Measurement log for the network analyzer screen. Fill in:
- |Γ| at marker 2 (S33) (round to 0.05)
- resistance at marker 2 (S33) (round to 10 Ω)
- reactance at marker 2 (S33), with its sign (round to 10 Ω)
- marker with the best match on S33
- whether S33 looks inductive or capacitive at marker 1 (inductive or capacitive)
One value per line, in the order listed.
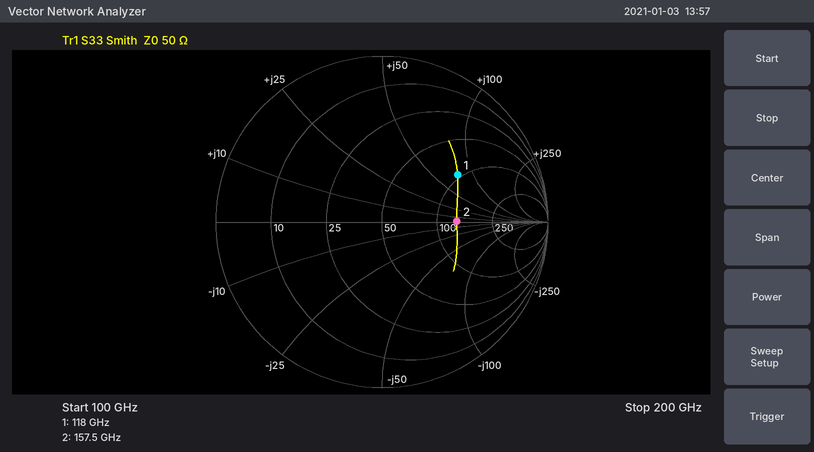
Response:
0.45
130 Ω
0 Ω
marker 2
inductive
